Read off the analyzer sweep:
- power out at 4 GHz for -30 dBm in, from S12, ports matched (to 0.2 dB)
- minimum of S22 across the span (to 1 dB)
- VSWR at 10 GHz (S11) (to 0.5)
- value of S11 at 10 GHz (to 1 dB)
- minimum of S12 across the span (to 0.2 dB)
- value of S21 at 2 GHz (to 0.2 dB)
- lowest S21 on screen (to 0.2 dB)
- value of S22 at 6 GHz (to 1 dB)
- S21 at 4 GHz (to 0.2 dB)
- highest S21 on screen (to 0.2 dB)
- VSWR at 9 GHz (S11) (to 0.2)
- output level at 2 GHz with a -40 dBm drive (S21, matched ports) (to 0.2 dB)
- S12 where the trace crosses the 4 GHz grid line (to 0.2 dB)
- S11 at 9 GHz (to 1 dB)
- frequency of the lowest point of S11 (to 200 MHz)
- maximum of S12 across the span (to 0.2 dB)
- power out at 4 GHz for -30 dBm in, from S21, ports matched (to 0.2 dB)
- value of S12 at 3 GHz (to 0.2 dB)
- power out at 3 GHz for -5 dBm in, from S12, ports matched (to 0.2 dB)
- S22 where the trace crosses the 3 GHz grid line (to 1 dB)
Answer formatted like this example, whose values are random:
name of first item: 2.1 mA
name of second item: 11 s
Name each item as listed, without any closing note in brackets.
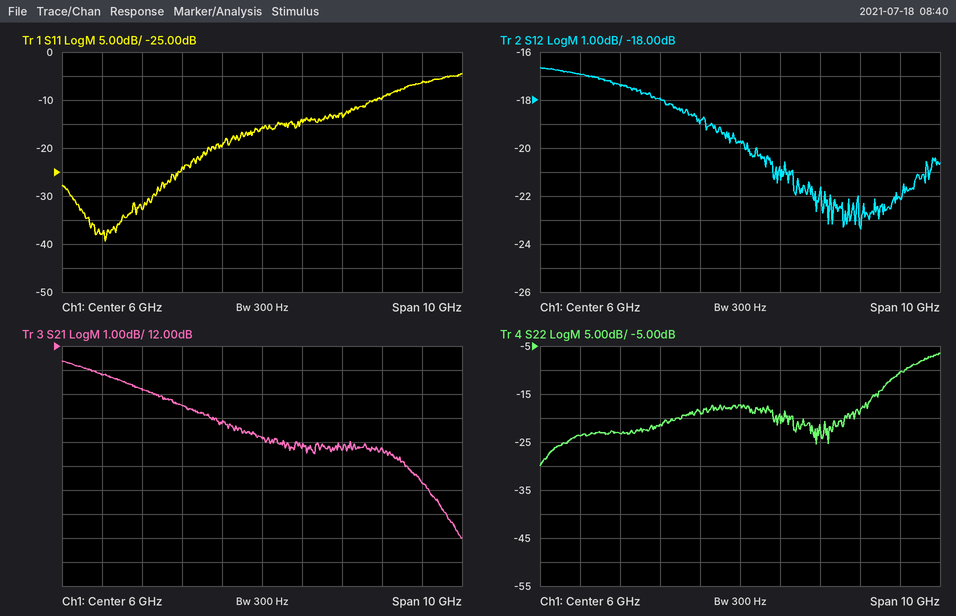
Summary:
power out at 4 GHz for -30 dBm in, from S12, ports matched: -48.0 dBm
minimum of S22 across the span: -30 dB
VSWR at 10 GHz (S11): 3.0
value of S11 at 10 GHz: -6 dB
minimum of S12 across the span: -23.4 dB
value of S21 at 2 GHz: 10.8 dB
lowest S21 on screen: 4.0 dB
value of S22 at 6 GHz: -17 dB
S21 at 4 GHz: 9.6 dB
highest S21 on screen: 11.4 dB
VSWR at 9 GHz (S11): 2.0
output level at 2 GHz with a -40 dBm drive (S21, matched ports): -29.2 dBm
S12 where the trace crosses the 4 GHz grid line: -18.0 dB
S11 at 9 GHz: -10 dB
frequency of the lowest point of S11: 2.0 GHz
maximum of S12 across the span: -16.6 dB
power out at 4 GHz for -30 dBm in, from S21, ports matched: -20.4 dBm
value of S12 at 3 GHz: -17.4 dB
power out at 3 GHz for -5 dBm in, from S12, ports matched: -22.4 dBm
S22 where the trace crosses the 3 GHz grid line: -23 dB
